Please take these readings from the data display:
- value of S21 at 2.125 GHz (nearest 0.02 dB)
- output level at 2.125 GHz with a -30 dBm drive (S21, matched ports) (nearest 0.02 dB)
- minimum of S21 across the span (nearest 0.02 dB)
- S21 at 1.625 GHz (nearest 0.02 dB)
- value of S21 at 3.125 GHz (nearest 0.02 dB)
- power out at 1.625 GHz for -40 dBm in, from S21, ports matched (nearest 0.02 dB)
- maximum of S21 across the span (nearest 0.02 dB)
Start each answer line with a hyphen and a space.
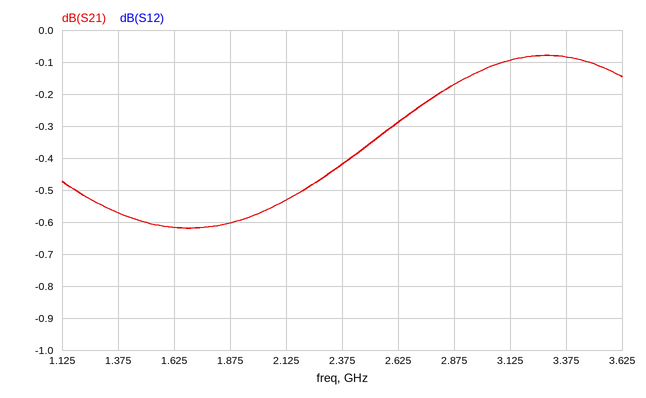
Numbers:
- -0.54 dB
- -30.54 dBm
- -0.62 dB
- -0.62 dB
- -0.10 dB
- -40.62 dBm
- -0.08 dB
